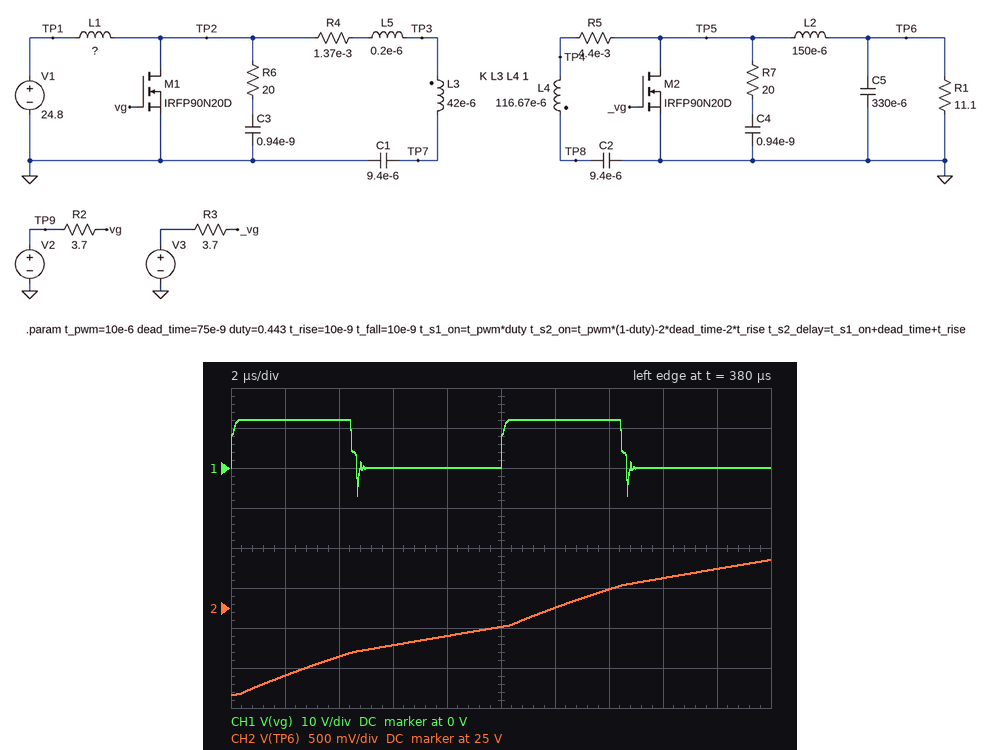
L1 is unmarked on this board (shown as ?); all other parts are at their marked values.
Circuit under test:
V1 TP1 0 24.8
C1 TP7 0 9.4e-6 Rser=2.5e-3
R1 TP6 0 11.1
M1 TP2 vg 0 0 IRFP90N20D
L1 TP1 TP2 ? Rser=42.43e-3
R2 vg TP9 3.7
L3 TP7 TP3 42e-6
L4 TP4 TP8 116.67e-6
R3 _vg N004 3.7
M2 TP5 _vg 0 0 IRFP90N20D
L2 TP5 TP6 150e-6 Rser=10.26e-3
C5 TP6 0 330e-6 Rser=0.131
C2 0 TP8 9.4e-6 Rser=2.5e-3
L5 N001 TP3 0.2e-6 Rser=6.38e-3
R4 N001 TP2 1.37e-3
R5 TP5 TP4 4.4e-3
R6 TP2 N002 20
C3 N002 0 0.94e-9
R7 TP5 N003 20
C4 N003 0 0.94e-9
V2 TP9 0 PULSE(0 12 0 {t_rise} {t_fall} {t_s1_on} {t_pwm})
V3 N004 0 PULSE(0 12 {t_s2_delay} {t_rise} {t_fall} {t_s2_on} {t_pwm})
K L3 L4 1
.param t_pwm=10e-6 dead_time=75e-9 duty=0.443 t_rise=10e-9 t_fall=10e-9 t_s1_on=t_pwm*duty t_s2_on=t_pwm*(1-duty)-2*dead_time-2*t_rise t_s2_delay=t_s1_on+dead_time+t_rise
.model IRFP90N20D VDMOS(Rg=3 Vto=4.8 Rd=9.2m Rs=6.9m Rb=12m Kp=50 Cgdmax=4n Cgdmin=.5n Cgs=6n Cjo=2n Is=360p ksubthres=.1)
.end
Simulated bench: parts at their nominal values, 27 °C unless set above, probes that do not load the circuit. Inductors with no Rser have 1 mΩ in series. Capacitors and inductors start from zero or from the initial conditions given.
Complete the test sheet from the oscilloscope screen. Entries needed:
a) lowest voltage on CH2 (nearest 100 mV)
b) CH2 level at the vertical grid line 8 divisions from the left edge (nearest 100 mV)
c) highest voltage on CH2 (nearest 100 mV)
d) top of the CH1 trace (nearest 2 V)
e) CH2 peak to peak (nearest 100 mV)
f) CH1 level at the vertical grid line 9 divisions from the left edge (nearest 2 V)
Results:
23.9 V
25.4 V
25.6 V
12 V
1.7 V
0 V
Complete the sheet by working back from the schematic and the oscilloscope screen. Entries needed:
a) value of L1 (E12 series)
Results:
39 µH
